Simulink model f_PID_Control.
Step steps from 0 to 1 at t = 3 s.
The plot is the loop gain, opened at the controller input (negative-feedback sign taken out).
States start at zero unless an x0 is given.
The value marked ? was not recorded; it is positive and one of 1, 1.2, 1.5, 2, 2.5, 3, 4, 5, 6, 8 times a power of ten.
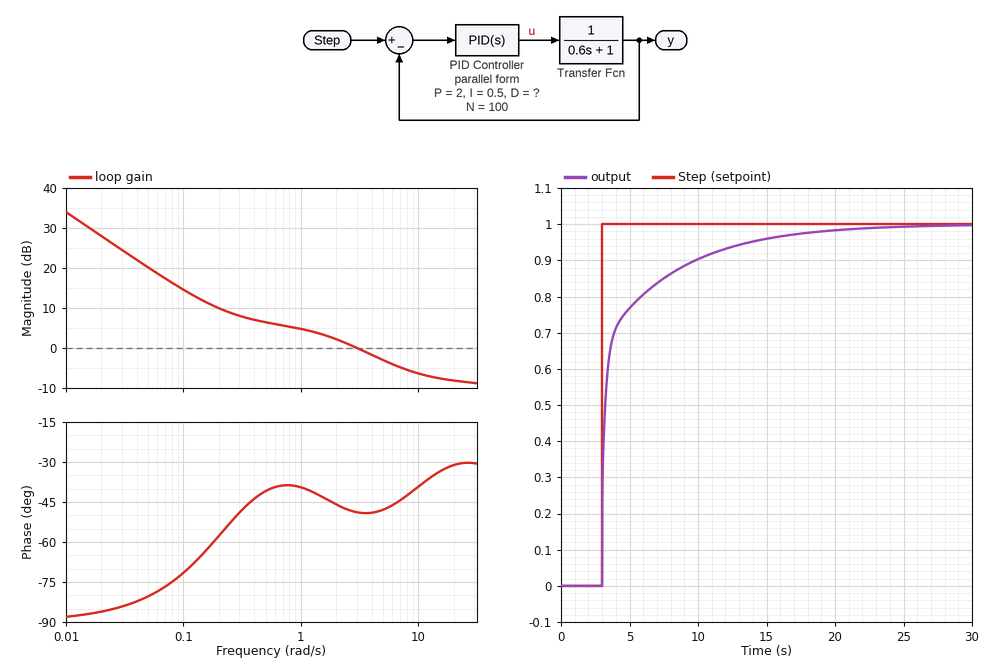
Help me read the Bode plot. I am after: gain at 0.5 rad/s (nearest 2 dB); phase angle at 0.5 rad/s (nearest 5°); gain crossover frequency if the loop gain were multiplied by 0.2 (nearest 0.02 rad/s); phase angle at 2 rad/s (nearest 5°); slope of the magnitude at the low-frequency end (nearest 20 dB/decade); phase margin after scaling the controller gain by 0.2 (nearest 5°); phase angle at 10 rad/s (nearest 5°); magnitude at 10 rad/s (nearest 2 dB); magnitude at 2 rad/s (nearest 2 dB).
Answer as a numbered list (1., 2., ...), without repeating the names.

1. 6 dB
2. -40°
3. 0.10 rad/s
4. -45°
5. -20 dB/decade
6. 110°
7. -40°
8. -6 dB
9. 2 dB
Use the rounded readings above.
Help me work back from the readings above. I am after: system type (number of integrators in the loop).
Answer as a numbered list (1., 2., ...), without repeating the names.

1. 1
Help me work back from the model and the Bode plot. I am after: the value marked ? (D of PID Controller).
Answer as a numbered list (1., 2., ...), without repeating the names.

1. 0.2
